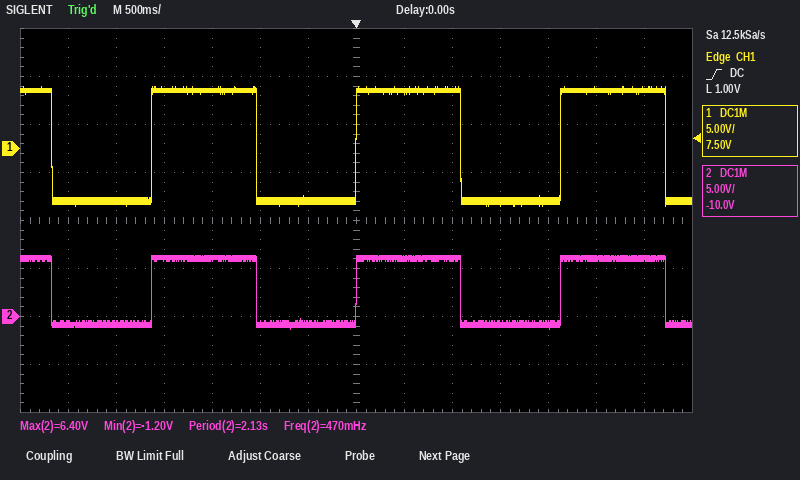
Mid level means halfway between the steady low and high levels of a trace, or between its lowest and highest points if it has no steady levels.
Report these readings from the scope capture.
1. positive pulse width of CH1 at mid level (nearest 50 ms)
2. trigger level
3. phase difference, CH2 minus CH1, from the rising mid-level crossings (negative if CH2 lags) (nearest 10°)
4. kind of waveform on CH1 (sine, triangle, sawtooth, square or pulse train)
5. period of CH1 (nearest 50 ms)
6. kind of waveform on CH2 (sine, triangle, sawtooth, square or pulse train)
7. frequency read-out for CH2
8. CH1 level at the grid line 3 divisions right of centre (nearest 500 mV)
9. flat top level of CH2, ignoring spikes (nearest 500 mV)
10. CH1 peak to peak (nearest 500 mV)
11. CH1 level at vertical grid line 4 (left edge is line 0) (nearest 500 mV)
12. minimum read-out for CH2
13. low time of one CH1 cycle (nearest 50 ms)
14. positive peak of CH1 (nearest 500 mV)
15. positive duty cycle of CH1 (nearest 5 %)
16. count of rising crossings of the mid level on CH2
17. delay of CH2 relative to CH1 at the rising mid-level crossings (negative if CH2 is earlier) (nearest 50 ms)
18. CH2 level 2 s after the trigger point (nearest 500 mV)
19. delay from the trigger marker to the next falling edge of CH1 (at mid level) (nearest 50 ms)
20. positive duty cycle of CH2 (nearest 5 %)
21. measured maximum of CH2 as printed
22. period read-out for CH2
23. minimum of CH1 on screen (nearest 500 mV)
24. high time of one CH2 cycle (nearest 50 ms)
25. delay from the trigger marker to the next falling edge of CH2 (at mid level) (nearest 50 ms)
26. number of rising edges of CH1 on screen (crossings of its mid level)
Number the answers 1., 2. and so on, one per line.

1. 1.10 s
2. 1.00 V
3. 0°
4. square
5. 2.15 s
6. square
7. 470 mHz
8. -5.5 V
9. 6.0 V
10. 12.5 V
11. 6.0 V
12. -1.20 V
13. 1.05 s
14. 6.5 V
15. 50 %
16. 3
17. 0 ms
18. -1.0 V
19. 1.10 s
20. 50 %
21. 6.40 V
22. 2.13 s
23. -6.0 V
24. 1.10 s
25. 1.10 s
26. 3
